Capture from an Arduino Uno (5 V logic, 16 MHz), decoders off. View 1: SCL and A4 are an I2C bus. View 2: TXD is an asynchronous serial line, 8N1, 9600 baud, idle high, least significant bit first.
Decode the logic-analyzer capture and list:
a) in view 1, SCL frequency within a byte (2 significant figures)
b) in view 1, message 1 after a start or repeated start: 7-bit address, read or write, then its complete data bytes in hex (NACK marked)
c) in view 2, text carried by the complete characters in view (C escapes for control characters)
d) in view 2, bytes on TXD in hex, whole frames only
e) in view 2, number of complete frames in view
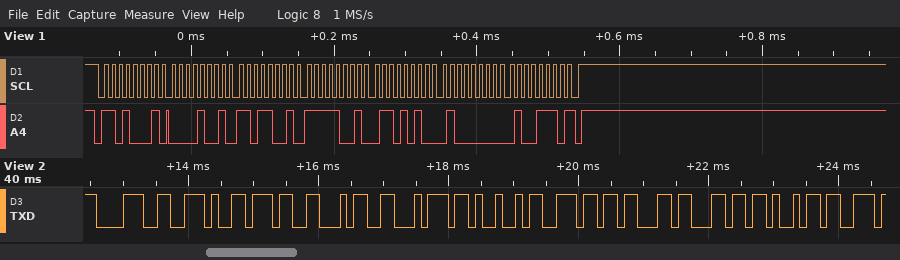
100 kHz
0x68 read: 09 D9 F9 6A 40 4E NACK
"8.74tIncli"
38 2E 37 34 74 49 6E 63 6C 69
10
